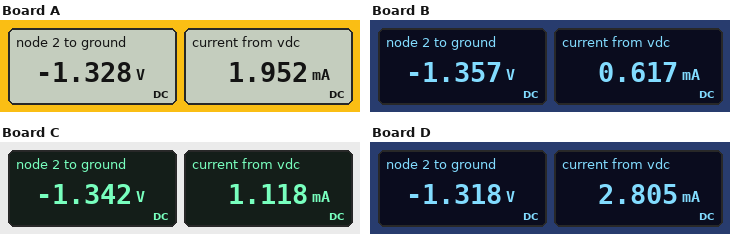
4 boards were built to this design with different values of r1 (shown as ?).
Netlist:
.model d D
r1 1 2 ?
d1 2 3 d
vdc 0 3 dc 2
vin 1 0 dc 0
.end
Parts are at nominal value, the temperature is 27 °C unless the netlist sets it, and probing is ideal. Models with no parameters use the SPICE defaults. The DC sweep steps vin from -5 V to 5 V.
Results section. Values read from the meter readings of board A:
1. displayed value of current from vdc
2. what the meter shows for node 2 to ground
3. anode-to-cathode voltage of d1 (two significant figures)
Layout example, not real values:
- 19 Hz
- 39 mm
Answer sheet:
- 1.952 mA
- -1.328 V
- 670 mV
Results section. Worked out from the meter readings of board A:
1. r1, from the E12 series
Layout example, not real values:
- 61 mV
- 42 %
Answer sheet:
- 680 Ω
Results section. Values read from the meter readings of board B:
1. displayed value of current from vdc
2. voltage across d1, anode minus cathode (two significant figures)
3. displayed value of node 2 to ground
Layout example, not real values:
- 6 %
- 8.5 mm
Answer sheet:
- 0.617 mA
- 640 mV
- -1.357 V
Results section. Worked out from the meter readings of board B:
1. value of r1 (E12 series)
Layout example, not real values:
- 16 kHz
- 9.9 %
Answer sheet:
- 2.2 kΩ
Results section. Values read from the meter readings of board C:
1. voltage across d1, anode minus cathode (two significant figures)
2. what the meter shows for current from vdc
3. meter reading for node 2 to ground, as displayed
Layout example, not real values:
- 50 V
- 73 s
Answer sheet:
- 660 mV
- 1.118 mA
- -1.342 V
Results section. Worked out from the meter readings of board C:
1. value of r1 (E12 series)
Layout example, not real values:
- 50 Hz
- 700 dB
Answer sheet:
- 1.2 kΩ
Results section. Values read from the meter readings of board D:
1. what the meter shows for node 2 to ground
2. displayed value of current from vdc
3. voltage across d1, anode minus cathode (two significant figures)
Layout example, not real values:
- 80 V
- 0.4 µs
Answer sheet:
- -1.318 V
- 2.805 mA
- 680 mV
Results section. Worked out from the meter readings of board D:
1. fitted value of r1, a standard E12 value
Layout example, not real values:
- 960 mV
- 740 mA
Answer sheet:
- 470 Ω
